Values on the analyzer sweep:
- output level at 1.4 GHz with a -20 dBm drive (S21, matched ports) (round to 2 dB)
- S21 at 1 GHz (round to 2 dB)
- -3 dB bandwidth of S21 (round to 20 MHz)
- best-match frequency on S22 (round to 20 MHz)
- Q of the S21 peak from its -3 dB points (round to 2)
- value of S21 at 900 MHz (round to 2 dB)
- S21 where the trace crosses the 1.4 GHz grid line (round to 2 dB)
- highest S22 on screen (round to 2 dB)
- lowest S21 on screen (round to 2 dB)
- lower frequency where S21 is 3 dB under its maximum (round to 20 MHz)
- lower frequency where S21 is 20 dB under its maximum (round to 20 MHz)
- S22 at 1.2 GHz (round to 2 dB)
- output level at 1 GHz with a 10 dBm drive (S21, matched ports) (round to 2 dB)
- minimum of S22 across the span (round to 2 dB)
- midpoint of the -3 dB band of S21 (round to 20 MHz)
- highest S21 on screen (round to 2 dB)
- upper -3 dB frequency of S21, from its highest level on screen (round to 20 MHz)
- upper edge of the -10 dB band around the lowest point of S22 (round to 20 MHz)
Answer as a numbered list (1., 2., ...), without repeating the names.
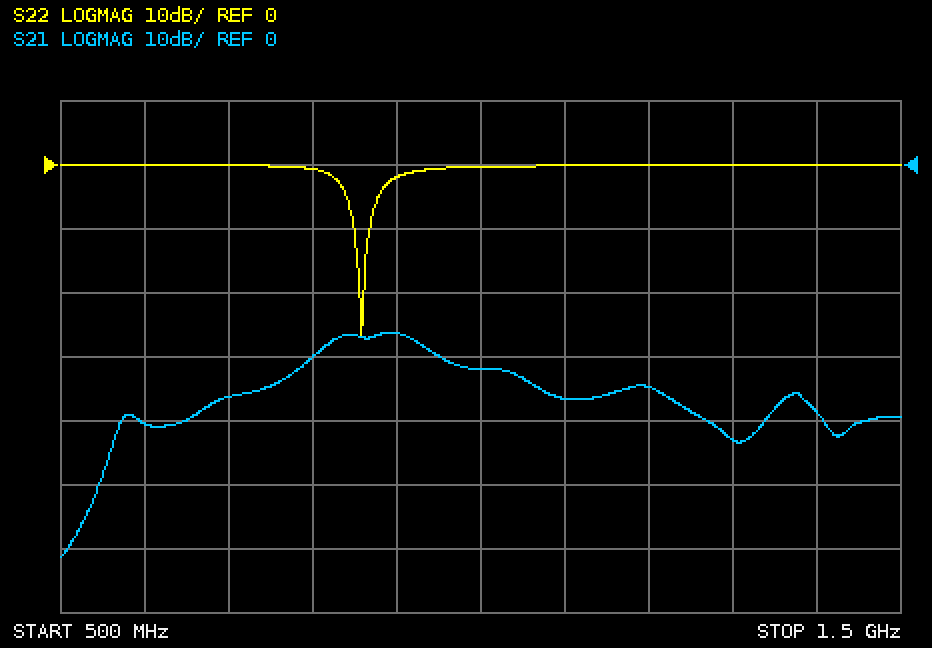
1. -58 dBm
2. -32 dB
3. 140 MHz
4. 860 MHz
5. 6
6. -26 dB
7. -38 dB
8. 0 dB
9. -62 dB
10. 800 MHz
11. 560 MHz
12. 0 dB
13. -22 dBm
14. -26 dB
15. 880 MHz
16. -26 dB
17. 940 MHz
18. 860 MHz
